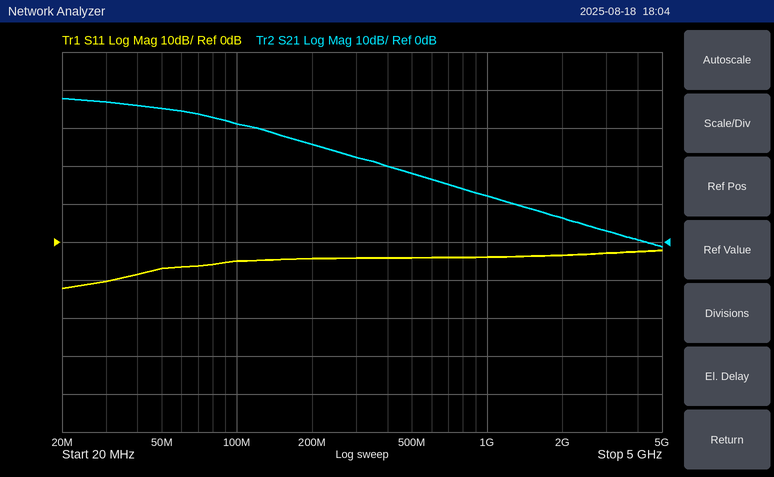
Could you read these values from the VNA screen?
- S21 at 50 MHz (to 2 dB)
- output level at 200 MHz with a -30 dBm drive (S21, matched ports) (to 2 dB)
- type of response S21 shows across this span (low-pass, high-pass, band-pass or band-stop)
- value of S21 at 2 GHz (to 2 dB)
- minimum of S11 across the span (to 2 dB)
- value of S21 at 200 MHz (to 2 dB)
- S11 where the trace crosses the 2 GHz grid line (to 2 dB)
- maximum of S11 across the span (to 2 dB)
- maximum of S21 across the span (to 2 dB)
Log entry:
36 dB
-4 dBm
low-pass
6 dB
-12 dB
26 dB
-4 dB
-2 dB
38 dB
